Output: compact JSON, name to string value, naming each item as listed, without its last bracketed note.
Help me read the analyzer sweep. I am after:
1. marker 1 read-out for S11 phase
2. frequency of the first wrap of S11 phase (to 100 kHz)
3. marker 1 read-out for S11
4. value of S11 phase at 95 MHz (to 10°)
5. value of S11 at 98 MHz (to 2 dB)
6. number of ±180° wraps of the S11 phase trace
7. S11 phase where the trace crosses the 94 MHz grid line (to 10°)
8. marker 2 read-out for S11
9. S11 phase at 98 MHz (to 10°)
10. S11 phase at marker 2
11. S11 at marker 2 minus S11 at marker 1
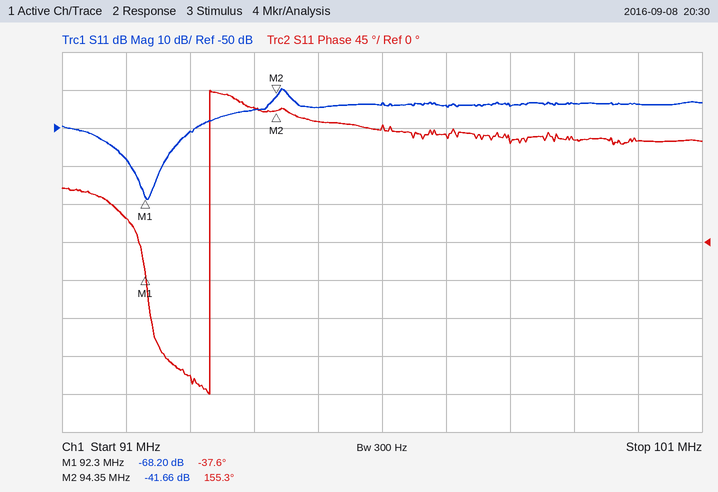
{"marker 1 read-out for S11 phase": "-37.6°", "frequency of the first wrap of S11 phase": "93.3 MHz", "marker 1 read-out for S11": "-68.20 dB", "value of S11 phase at 95 MHz": "140°", "value of S11 at 98 MHz": "-44 dB", "number of ±180° wraps of the S11 phase trace": "1", "S11 phase where the trace crosses the 94 MHz grid line": "160°", "marker 2 read-out for S11": "-41.66 dB", "S11 phase at 98 MHz": "120°", "S11 phase at marker 2": "155.3°", "S11 at marker 2 minus S11 at marker 1": "26.54 dB"}
